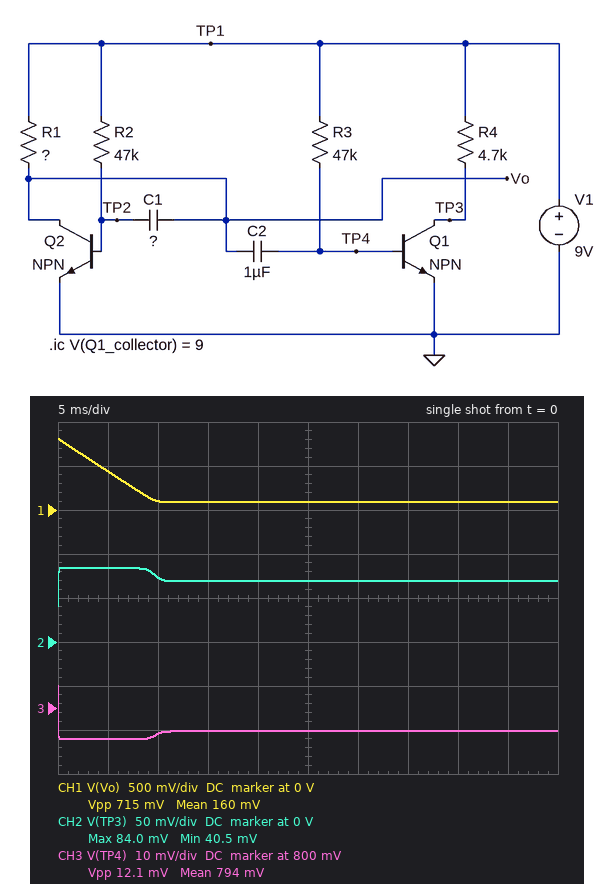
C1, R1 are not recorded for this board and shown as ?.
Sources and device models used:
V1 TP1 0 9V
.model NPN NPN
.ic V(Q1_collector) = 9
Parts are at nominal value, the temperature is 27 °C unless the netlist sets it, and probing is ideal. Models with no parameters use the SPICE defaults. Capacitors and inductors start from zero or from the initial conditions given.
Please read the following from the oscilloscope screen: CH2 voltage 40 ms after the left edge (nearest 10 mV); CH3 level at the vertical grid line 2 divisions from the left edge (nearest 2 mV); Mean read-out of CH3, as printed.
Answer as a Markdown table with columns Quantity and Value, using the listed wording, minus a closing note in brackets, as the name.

| Quantity | Value |
|---|---|
| CH2 voltage 40 ms after the left edge | 70 mV |
| CH3 level at the vertical grid line 2 divisions from the left edge | 794 mV |
| Mean read-out of CH3, as printed | 794 mV |
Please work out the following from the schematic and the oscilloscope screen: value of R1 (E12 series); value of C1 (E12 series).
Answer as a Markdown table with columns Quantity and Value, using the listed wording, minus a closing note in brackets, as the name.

| Quantity | Value |
|---|---|
| value of R1 | 2.2 kΩ |
| value of C1 | 1.8 µF |
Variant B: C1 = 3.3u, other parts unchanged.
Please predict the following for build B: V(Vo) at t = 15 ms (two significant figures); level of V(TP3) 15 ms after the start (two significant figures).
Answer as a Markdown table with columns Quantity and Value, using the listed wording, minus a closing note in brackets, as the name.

| Quantity | Value |
|---|---|
| V(Vo) at t = 15 ms | 200 mV |
| level of V(TP3) 15 ms after the start | 76 mV |
